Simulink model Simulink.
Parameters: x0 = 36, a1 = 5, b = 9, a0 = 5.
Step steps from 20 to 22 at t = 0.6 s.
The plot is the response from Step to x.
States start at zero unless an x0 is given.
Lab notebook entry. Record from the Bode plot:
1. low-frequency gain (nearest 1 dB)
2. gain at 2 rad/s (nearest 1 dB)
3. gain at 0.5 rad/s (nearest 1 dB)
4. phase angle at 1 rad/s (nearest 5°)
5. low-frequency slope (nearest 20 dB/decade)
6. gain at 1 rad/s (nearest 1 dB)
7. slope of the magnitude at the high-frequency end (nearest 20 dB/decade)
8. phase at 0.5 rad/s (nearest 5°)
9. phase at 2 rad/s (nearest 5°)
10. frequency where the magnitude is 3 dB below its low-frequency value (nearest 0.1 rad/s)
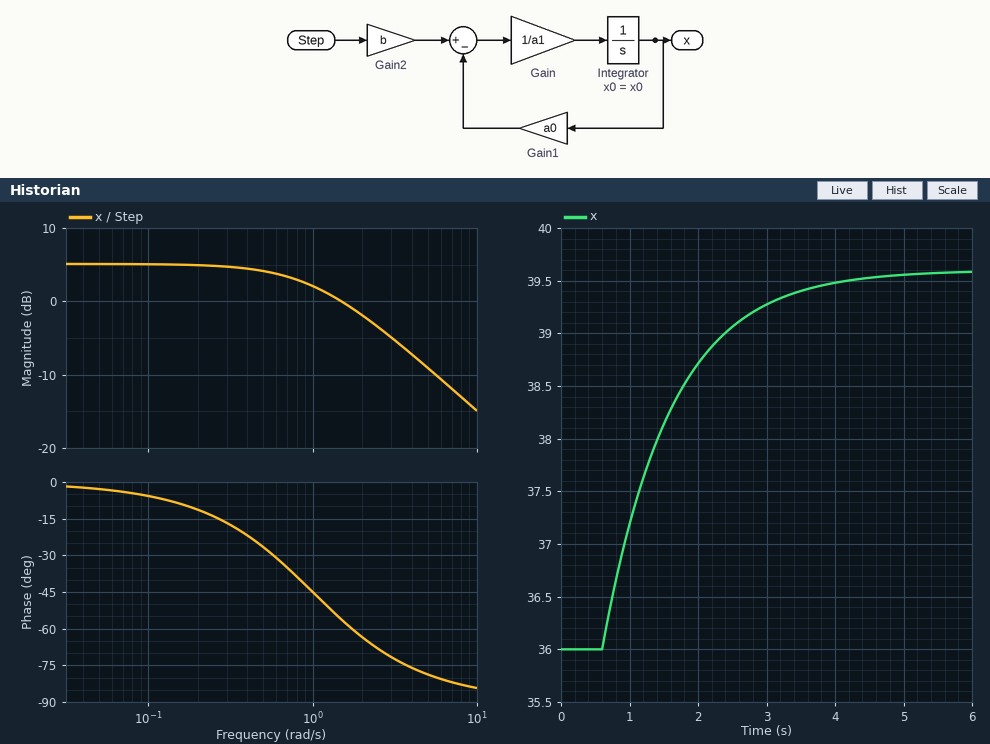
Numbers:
5 dB
-2 dB
4 dB
-45°
0 dB/decade
2 dB
-20 dB/decade
-25°
-65°
1.0 rad/s
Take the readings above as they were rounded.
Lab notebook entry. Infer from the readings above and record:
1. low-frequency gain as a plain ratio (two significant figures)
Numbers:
1.8
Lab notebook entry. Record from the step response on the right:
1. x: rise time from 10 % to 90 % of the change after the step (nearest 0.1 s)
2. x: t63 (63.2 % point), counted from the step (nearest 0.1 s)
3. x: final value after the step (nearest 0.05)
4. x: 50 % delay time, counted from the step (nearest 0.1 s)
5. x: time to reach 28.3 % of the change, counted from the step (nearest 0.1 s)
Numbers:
2.2 s
1.0 s
39.60
0.7 s
0.3 s
